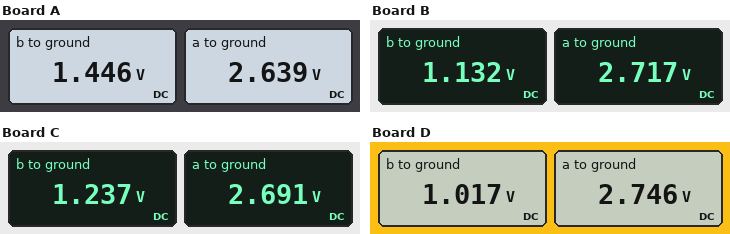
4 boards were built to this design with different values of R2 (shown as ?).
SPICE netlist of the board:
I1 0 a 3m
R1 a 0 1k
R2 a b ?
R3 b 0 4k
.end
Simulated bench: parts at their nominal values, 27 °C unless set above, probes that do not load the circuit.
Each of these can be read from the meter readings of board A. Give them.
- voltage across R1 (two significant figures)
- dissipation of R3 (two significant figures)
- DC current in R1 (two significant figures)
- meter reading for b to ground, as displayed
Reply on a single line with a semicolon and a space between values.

2.6 V; 520 µW; 2.6 mA; 1.446 V
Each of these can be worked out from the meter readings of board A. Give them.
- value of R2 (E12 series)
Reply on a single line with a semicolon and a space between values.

3.3 kΩ
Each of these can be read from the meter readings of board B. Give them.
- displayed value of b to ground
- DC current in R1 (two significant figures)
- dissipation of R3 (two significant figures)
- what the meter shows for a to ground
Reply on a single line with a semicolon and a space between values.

1.132 V; 2.7 mA; 320 µW; 2.717 V
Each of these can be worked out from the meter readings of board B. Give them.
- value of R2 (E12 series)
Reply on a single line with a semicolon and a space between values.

5.6 kΩ
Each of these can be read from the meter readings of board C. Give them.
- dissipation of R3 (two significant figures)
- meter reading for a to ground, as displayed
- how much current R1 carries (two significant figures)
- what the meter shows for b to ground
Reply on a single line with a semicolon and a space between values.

380 µW; 2.691 V; 2.7 mA; 1.237 V
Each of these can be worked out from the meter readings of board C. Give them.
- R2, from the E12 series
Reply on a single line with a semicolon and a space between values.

4.7 kΩ
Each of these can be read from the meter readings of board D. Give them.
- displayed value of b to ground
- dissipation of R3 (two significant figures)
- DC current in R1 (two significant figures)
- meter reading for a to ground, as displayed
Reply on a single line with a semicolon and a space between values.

1.017 V; 260 µW; 2.7 mA; 2.746 V
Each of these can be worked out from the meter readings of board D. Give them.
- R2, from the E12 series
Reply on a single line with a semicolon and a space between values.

6.8 kΩ
